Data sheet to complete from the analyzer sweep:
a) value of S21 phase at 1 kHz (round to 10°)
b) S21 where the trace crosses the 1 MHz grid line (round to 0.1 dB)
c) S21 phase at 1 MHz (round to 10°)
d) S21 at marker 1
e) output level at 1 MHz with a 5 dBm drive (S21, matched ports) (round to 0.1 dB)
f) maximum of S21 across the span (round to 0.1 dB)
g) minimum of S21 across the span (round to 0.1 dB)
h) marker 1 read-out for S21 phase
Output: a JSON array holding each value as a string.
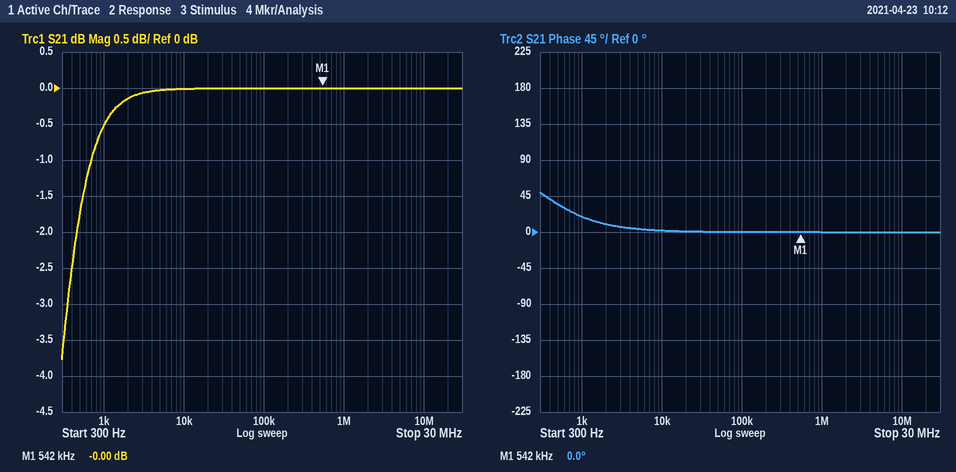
["20°", "0.0 dB", "0°", "-0.00 dB", "5.0 dBm", "0.0 dB", "-3.8 dB", "0.0°"]
